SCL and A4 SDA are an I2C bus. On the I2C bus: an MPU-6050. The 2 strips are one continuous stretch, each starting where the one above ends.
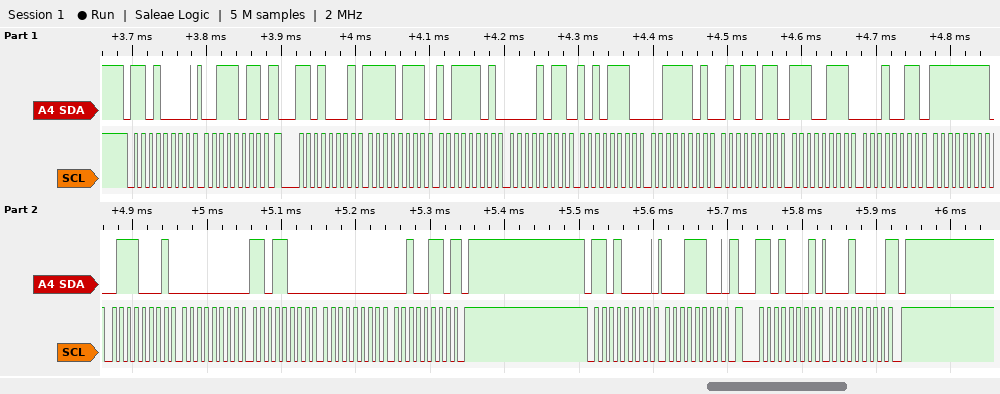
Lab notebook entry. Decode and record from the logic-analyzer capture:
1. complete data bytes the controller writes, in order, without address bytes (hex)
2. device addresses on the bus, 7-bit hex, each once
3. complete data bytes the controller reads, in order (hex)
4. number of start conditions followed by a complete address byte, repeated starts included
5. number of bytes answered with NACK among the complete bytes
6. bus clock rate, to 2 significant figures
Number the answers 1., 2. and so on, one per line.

1. 3B 1C
2. 0x68
3. F7 BD 0B AE 3D 5B E7 13 FF 71 00 D8 00 26 10
4. 4
5. 2
6. 100 kHz
